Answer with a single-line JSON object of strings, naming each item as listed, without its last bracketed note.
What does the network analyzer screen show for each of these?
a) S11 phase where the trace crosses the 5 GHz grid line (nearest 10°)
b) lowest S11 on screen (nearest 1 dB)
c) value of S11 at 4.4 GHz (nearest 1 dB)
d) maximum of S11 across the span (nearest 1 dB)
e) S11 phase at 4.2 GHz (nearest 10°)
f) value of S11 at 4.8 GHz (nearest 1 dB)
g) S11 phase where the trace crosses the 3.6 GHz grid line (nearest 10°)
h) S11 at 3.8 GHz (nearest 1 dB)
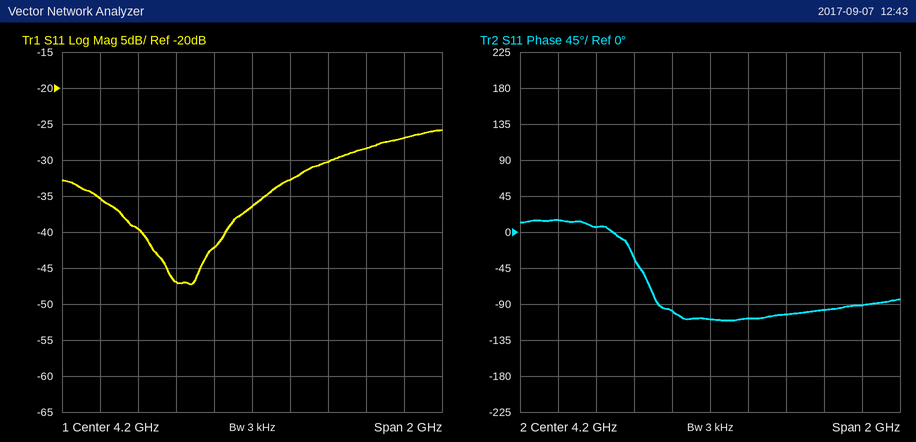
{"S11 phase where the trace crosses the 5 GHz grid line": "-90°", "lowest S11 on screen": "-47 dB", "value of S11 at 4.4 GHz": "-33 dB", "maximum of S11 across the span": "-26 dB", "S11 phase at 4.2 GHz": "-110°", "value of S11 at 4.8 GHz": "-28 dB", "S11 phase where the trace crosses the 3.6 GHz grid line": "10°", "S11 at 3.8 GHz": "-47 dB"}
